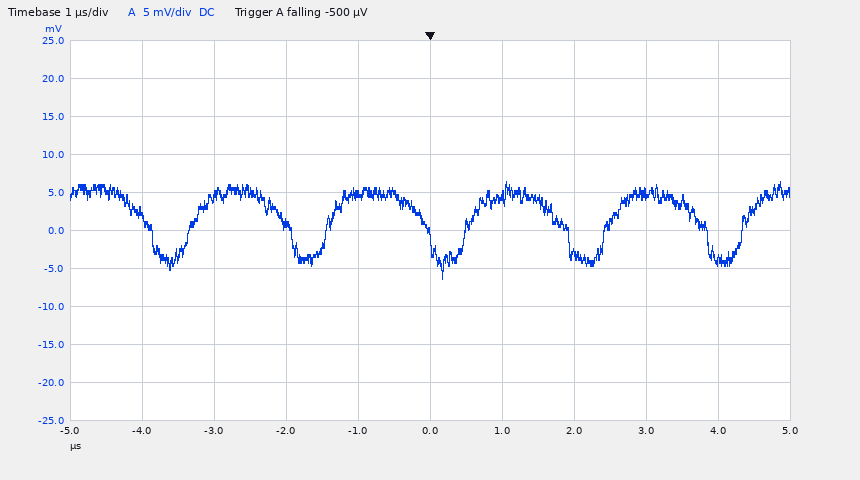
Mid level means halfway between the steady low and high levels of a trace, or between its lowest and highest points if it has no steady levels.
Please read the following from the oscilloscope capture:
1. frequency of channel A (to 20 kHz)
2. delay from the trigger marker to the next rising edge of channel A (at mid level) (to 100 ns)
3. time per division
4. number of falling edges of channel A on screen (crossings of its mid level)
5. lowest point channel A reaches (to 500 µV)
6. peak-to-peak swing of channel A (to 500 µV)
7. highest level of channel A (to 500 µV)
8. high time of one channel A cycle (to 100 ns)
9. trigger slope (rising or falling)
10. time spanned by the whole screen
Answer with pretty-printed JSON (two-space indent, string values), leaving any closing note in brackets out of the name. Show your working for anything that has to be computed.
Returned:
{
  "frequency of channel A": "520 kHz",
  "delay from the trigger marker to the next rising edge of channel A (at mid level)": "500 ns",
  "time per division": "1 µs",
  "number of falling edges of channel A on screen": "5",
  "lowest point channel A reaches": "-6.5 mV",
  "peak-to-peak swing of channel A": "6.5 mV − (-6.5 mV) = 13.0 mV",
  "highest level of channel A": "6.5 mV",
  "high time of one channel A cycle": "1.4 µs",
  "trigger slope": "falling",
  "time spanned by the whole screen": "10 µs"
}
